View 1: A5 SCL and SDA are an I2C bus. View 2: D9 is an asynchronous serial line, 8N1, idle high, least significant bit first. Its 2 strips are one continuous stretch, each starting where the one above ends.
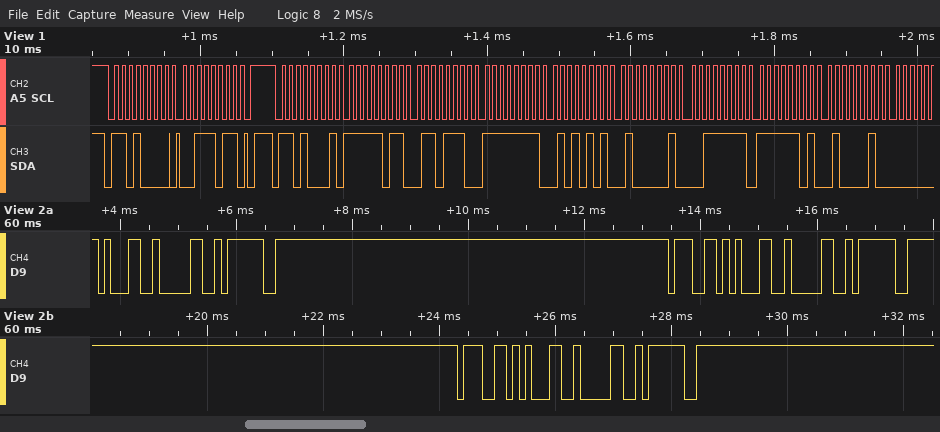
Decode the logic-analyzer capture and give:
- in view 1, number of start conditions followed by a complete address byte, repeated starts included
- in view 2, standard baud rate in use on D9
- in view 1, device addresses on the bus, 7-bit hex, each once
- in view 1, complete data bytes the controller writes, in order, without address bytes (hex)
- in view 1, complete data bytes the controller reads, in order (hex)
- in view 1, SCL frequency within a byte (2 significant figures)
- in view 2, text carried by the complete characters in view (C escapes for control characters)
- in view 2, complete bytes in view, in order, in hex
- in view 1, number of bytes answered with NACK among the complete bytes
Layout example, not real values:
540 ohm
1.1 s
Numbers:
2
9600 baud
0x68
3B
FB 6E FF 55 41 3F FD 42
100 kHz
"10?g10?g10?"
31 30 3F 67 31 30 3F 67 31 30 3F
0
